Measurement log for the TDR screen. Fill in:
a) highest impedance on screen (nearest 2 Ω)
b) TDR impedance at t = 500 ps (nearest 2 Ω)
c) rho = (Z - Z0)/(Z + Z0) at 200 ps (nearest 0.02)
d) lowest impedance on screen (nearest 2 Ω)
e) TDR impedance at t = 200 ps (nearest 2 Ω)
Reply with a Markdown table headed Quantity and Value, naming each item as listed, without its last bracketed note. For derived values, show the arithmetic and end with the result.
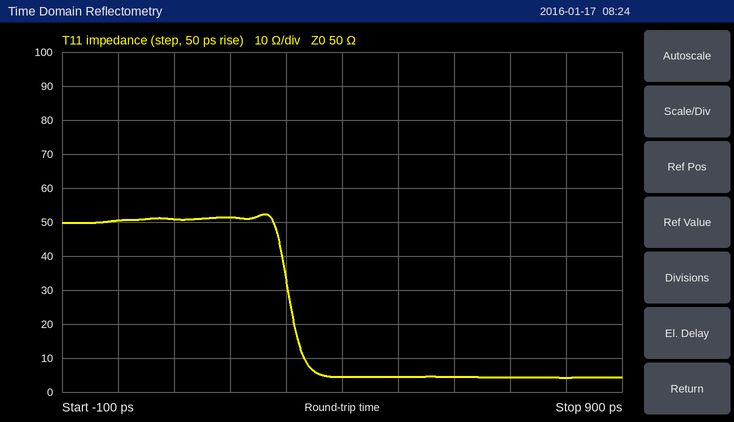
| Quantity | Value |
|---|---|
| highest impedance on screen | 52 Ω |
| TDR impedance at t = 500 ps | 4 Ω |
| rho = (Z - Z0)/(Z + Z0) at 200 ps | (52 − 50)/(52 + 50) ≈ +0.02 |
| lowest impedance on screen | 4 Ω |
| TDR impedance at t = 200 ps | 52 Ω |
